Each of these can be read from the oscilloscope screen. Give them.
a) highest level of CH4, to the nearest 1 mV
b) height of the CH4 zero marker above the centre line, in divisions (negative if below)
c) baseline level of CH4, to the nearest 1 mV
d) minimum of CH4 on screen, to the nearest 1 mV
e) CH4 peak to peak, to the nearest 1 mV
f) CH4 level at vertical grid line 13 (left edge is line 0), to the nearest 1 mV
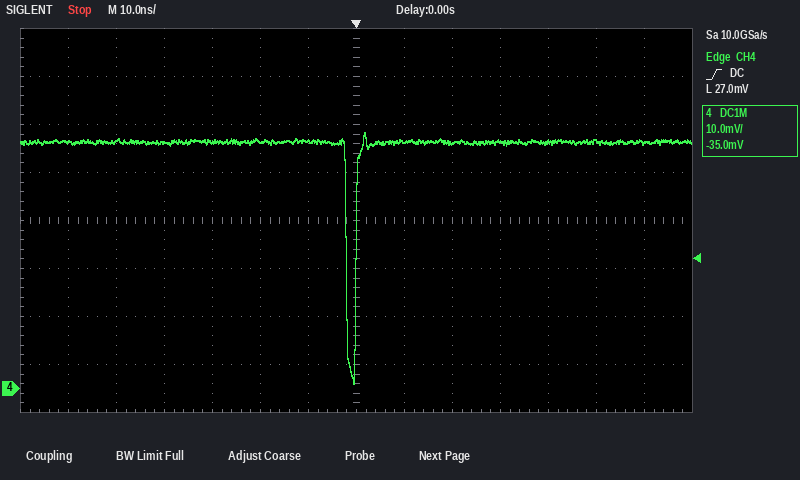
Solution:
53 mV
-3.5 div
51 mV
1 mV
52 mV
51 mV
